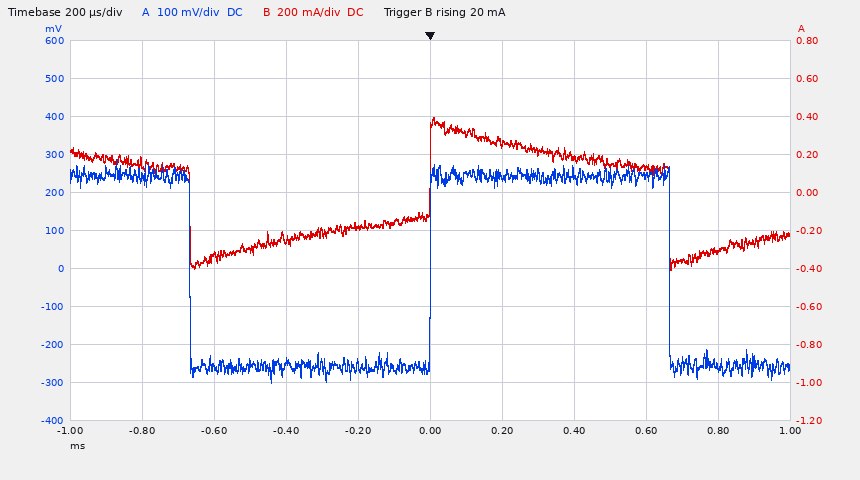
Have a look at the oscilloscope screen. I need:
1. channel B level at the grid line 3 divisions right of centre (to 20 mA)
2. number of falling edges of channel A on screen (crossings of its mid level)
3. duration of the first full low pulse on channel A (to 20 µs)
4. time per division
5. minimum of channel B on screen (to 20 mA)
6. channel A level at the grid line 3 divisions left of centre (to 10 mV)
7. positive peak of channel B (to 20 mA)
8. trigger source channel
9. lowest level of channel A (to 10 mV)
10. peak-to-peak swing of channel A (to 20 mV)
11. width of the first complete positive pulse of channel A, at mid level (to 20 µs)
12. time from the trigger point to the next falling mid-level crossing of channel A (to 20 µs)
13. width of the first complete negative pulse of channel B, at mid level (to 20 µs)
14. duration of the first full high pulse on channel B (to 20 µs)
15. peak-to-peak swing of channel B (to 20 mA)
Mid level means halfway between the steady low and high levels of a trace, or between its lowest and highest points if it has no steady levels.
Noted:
140 mA
2
660 µs
200 µs
-400 mA
-260 mV
400 mA
channel B
-300 mV
580 mV
660 µs
660 µs
660 µs
660 µs
800 mA
